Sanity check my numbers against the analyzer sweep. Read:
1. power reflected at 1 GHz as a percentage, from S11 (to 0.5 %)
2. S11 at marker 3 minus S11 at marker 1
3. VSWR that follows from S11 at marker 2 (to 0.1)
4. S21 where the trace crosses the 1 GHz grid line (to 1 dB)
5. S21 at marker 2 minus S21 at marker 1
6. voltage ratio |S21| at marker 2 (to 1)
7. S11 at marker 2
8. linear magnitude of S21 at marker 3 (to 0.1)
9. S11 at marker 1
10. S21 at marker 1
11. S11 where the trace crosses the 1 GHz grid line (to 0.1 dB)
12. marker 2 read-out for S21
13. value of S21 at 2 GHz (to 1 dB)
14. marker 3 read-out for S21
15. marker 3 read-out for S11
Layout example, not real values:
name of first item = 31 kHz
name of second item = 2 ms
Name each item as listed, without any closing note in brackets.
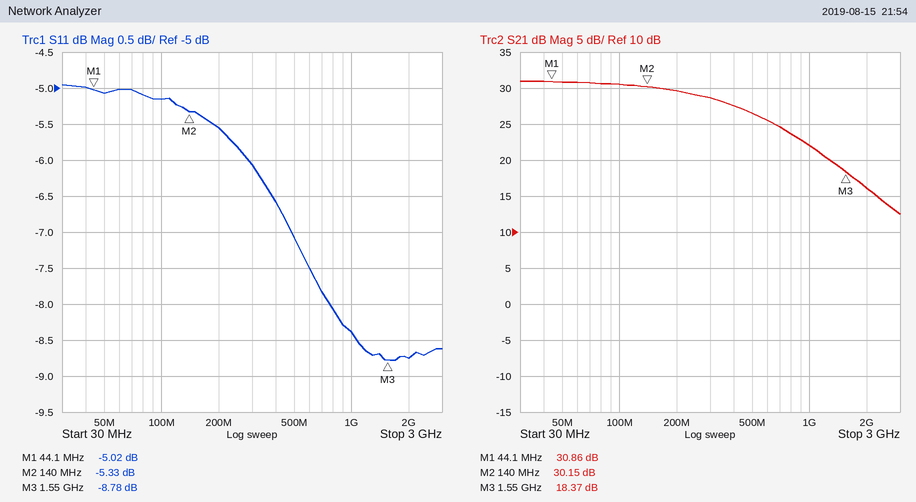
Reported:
power reflected at 1 GHz as a percentage, from S11 = 14.5 %
S11 at marker 3 minus S11 at marker 1 = -3.76 dB
VSWR that follows from S11 at marker 2 = 3.4
S21 where the trace crosses the 1 GHz grid line = 22 dB
S21 at marker 2 minus S21 at marker 1 = -0.71 dB
voltage ratio |S21| at marker 2 = 32
S11 at marker 2 = -5.33 dB
linear magnitude of S21 at marker 3 = 8.3
S11 at marker 1 = -5.02 dB
S21 at marker 1 = 30.86 dB
S11 where the trace crosses the 1 GHz grid line = -8.4 dB
marker 2 read-out for S21 = 30.15 dB
value of S21 at 2 GHz = 16 dB
marker 3 read-out for S21 = 18.37 dB
marker 3 read-out for S11 = -8.78 dB
